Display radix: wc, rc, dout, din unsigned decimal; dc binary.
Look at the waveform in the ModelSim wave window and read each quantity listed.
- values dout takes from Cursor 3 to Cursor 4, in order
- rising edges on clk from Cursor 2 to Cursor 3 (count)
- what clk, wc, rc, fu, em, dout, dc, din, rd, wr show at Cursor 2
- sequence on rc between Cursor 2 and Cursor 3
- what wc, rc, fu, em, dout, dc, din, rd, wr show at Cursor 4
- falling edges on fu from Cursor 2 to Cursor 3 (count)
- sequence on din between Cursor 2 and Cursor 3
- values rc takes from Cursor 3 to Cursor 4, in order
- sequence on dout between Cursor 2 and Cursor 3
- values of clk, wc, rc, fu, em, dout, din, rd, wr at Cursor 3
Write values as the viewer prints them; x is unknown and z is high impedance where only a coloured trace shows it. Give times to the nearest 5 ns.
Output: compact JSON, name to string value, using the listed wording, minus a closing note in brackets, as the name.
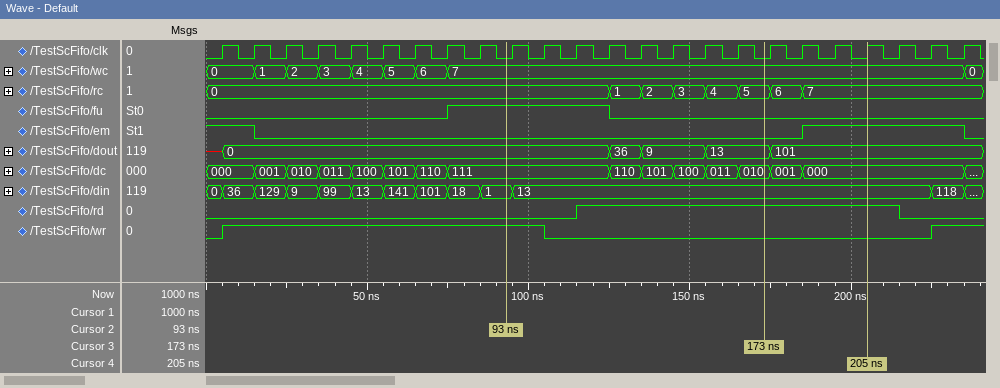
{"values dout takes from Cursor 3 to Cursor 4, in order": "13, 101", "rising edges on clk from Cursor 2 to Cursor 3": "8", "what clk, wc, rc, fu, em, dout, dc, din, rd, wr show at Cursor 2": "clk=0, wc=7, rc=0, fu=1, em=0, dout=0, dc=111, din=1, rd=0, wr=1", "sequence on rc between Cursor 2 and Cursor 3": "0, 1, 2, 3, 4, 5", "what wc, rc, fu, em, dout, dc, din, rd, wr show at Cursor 4": "wc=7, rc=7, fu=0, em=1, dout=101, dc=000, din=13, rd=1, wr=0", "falling edges on fu from Cursor 2 to Cursor 3": "1", "sequence on din between Cursor 2 and Cursor 3": "1, 13", "values rc takes from Cursor 3 to Cursor 4, in order": "5, 6, 7", "sequence on dout between Cursor 2 and Cursor 3": "0, 36, 9, 13", "values of clk, wc, rc, fu, em, dout, din, rd, wr at Cursor 3": "clk=0, wc=7, rc=5, fu=0, em=0, dout=13, din=13, rd=1, wr=0"}
